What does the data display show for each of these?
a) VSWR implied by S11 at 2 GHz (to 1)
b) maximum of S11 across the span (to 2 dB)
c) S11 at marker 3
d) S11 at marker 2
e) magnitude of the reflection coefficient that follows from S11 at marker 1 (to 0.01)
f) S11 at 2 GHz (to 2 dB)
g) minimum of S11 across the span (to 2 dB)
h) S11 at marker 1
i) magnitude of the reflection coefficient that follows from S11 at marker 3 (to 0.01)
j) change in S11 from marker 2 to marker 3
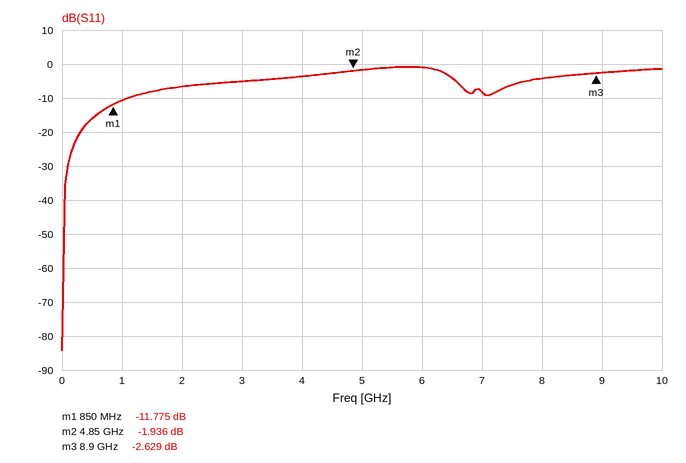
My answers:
3
0 dB
-2.629 dB
-1.936 dB
0.26
-6 dB
-84 dB
-11.775 dB
0.74
-0.693 dB
